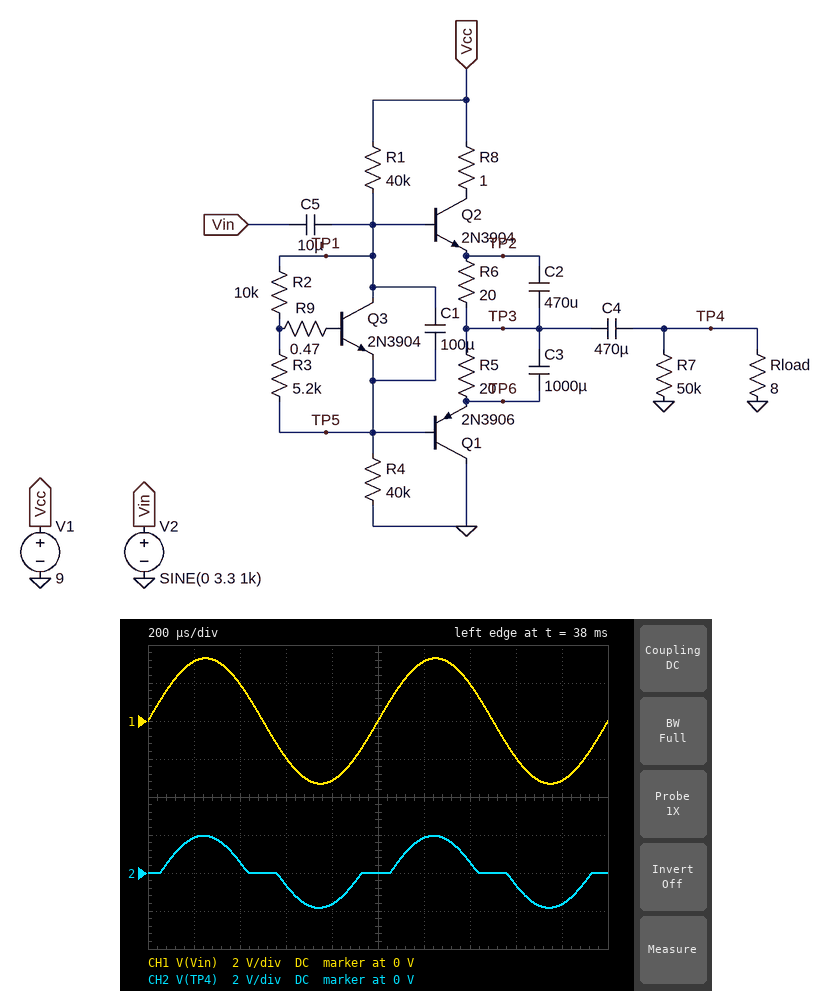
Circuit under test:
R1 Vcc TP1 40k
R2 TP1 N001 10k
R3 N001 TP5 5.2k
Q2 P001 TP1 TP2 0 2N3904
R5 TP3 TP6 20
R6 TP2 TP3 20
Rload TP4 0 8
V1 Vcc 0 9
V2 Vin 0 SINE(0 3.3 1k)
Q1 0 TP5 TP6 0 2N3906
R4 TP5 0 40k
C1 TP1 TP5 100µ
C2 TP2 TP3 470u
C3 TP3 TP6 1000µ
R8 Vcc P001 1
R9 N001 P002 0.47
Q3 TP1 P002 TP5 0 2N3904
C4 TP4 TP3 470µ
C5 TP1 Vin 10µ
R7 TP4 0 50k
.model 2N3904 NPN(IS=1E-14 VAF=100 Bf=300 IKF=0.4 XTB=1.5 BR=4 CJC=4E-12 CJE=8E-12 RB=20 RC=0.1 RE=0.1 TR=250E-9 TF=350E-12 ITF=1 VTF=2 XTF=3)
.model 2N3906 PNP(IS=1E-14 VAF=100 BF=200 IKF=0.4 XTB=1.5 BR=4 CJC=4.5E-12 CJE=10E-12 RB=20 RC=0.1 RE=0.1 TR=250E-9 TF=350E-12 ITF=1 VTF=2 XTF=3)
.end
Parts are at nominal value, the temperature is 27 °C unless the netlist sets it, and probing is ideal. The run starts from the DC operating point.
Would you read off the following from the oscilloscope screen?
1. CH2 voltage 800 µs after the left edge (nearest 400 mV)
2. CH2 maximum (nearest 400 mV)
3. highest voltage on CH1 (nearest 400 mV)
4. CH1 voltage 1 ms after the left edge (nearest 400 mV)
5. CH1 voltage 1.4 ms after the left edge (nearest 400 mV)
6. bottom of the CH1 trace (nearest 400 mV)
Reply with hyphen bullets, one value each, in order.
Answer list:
- -1.6 V
- 2.0 V
- 3.2 V
- 0 V
- 2.0 V
- -3.2 V
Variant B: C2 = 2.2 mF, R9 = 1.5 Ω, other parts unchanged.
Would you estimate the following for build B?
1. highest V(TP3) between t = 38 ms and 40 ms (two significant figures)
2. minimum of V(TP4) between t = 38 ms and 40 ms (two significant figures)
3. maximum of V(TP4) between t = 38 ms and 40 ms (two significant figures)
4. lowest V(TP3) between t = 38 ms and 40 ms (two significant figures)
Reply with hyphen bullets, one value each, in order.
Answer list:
- 7.2 V
- -1.9 V
- 2.0 V
- 3.2 V
